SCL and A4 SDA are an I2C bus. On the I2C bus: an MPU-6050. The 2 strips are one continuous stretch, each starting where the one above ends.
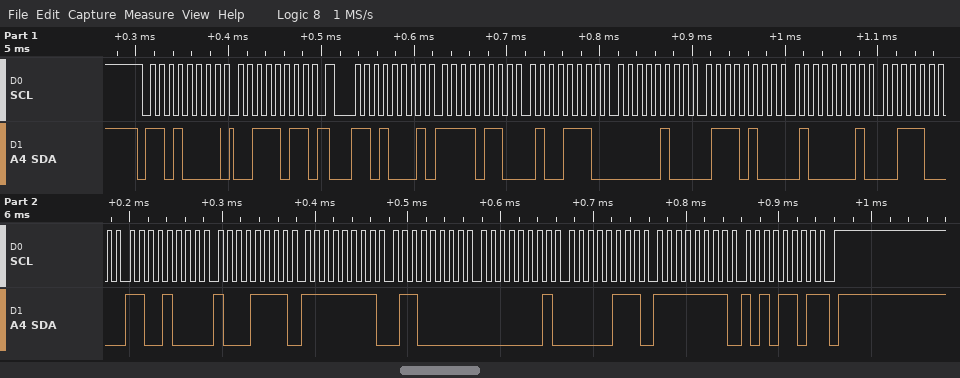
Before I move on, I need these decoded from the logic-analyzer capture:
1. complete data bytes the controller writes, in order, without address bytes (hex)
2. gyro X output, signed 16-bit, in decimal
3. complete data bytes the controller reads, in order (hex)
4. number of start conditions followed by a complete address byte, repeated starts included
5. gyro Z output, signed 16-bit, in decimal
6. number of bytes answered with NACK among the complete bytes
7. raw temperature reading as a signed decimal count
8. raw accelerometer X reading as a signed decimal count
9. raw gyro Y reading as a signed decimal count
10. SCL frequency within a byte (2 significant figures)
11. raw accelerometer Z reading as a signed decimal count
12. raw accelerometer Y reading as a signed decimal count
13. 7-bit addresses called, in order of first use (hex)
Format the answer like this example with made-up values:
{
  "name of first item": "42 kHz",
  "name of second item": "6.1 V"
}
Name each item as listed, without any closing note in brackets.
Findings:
{
  "complete data bytes the controller writes, in order, without address bytes": "3B",
  "gyro X output, signed 16-bit, in decimal": "-160",
  "complete data bytes the controller reads, in order": "F6 4E 04 74 41 38 C8 8F FF 60 01 07 FF AD",
  "number of start conditions followed by a complete address byte, repeated starts included": "2",
  "gyro Z output, signed 16-bit, in decimal": "-83",
  "number of bytes answered with NACK among the complete bytes": "1",
  "raw temperature reading as a signed decimal count": "-14193",
  "raw accelerometer X reading as a signed decimal count": "-2482",
  "raw gyro Y reading as a signed decimal count": "263",
  "SCL frequency within a byte": "100 kHz",
  "raw accelerometer Z reading as a signed decimal count": "16696",
  "raw accelerometer Y reading as a signed decimal count": "1140",
  "7-bit addresses called, in order of first use": "0x68"
}
